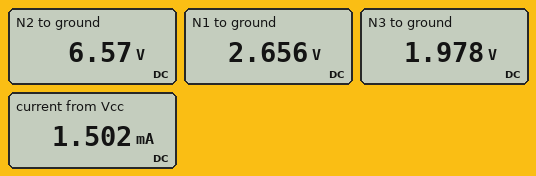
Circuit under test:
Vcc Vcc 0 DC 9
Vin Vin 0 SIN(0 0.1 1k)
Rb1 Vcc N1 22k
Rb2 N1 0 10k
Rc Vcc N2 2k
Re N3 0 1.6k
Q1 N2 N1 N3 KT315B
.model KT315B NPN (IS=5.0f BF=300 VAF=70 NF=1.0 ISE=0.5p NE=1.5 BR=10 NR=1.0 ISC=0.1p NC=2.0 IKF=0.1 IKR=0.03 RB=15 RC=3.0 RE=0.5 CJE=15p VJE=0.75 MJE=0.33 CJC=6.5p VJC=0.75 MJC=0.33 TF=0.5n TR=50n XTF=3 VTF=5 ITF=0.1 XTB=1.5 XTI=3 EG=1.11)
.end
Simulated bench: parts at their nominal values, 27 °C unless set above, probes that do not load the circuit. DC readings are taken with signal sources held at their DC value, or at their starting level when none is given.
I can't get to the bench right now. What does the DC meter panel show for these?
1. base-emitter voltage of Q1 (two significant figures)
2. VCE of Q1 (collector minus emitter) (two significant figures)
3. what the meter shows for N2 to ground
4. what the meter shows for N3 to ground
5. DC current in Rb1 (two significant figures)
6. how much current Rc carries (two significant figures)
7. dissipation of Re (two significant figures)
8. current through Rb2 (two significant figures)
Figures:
680 mV
4.6 V
6.57 V
1.978 V
290 µA
1.2 mA
2.4 mW
270 µA
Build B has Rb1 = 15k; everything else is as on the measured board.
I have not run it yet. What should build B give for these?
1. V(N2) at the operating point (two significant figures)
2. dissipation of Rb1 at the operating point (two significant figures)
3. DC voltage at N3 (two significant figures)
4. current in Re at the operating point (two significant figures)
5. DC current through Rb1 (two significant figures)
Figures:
5.6 V
2.1 mW
2.7 V
1.7 mA
370 µA
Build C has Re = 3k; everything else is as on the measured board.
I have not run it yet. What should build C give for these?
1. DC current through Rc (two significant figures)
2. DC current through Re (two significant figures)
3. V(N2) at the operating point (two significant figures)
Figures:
670 µA
680 µA
7.7 V
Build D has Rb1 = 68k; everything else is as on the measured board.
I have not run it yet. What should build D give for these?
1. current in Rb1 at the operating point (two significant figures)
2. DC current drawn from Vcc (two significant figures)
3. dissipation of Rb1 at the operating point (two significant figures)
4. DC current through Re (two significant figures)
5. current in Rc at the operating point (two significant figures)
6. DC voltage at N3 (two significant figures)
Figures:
120 µA
390 µA
920 µW
280 µA
270 µA
450 mV
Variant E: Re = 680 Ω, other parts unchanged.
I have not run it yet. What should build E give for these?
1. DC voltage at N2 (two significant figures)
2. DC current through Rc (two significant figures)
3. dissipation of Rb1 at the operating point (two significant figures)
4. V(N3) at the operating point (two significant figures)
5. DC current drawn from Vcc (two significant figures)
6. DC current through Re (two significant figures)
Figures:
3.7 V
2.6 mA
1.9 mW
1.8 V
2.9 mA
2.7 mA
